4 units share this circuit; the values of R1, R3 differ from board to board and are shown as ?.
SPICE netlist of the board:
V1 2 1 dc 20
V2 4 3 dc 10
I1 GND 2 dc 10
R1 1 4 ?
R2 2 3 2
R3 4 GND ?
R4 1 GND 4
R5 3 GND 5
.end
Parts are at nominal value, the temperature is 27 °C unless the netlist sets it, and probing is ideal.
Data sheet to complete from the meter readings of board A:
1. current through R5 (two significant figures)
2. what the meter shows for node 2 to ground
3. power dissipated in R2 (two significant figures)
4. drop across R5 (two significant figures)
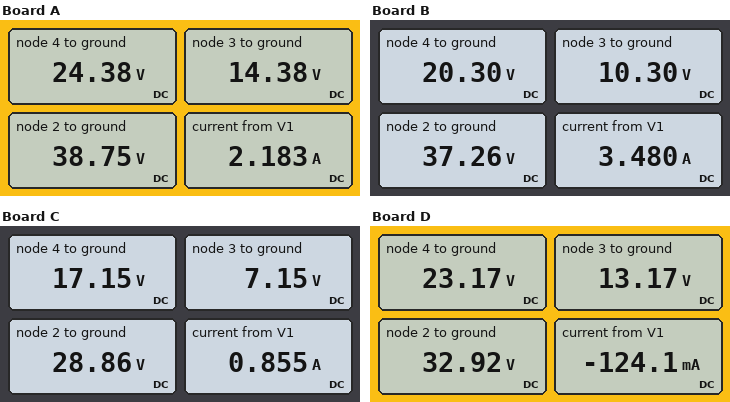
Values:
2.9 A
38.75 V
300 W
14 V
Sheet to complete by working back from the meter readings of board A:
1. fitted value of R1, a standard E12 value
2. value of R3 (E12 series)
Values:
0.82 Ω
10 Ω
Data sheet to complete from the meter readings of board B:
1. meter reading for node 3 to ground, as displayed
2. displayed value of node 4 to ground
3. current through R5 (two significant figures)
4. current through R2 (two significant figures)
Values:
10.30 V
20.30 V
2.1 A
13 A
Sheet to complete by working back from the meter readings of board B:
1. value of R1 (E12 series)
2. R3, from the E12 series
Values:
0.39 Ω
5.6 Ω
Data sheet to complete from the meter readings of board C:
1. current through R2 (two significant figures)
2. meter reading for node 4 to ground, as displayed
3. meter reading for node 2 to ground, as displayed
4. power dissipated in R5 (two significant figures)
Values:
11 A
17.15 V
28.86 V
10 W
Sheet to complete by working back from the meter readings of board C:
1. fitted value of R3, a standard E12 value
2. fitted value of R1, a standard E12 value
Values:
2.7 Ω
2.7 Ω
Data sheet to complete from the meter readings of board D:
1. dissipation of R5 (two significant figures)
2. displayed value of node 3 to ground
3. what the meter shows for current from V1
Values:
35 W
13.17 V
-124.1 mA
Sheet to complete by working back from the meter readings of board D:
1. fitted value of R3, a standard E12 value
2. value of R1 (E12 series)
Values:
5.6 Ω
3.3 Ω
